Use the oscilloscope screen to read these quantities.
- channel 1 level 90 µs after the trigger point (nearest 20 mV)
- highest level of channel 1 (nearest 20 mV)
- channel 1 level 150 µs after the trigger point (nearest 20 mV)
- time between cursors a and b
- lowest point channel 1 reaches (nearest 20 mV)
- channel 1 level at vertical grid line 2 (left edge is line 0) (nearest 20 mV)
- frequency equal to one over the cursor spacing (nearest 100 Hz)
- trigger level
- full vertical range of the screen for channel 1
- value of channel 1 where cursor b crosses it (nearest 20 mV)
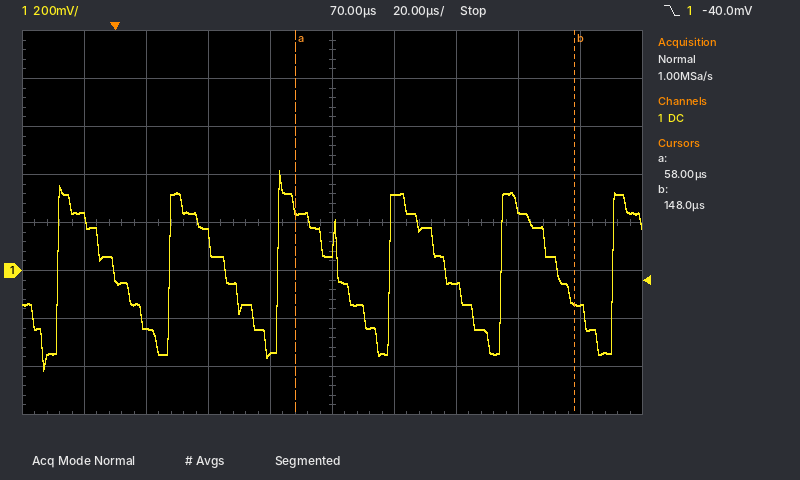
320 mV
420 mV
-140 mV
90 µs
-420 mV
-240 mV
11.1 kHz
-40.0 mV
1.6 V
-140 mV
